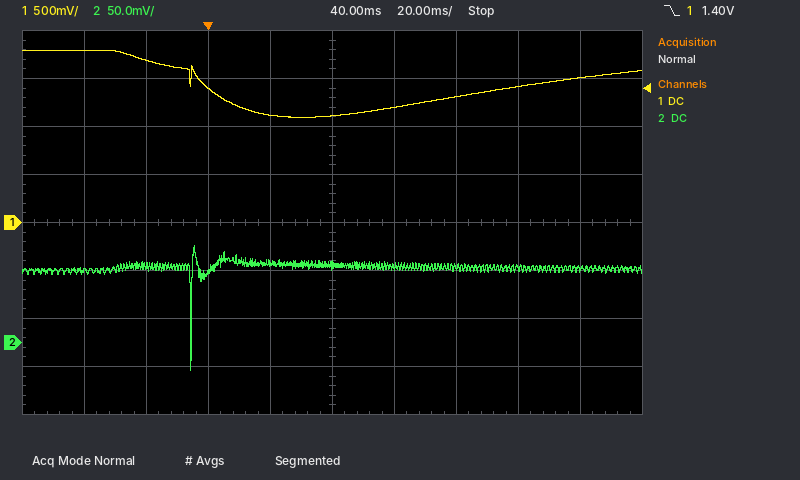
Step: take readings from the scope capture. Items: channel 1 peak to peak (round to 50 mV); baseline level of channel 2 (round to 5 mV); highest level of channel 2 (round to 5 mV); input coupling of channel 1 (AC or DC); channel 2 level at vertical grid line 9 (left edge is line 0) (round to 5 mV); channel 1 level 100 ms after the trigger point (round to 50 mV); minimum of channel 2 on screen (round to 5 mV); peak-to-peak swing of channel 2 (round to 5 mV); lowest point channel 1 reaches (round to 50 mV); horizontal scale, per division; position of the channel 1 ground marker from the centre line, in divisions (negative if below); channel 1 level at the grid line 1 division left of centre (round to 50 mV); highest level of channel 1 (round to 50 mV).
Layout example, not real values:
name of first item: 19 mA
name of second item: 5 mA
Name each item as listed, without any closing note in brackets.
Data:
channel 1 peak to peak: 700 mV
baseline level of channel 2: 80 mV
highest level of channel 2: 100 mV
input coupling of channel 1: DC
channel 2 level at vertical grid line 9 (left edge is line 0): 75 mV
channel 1 level 100 ms after the trigger point: 1.40 V
minimum of channel 2 on screen: -30 mV
peak-to-peak swing of channel 2: 130 mV
lowest point channel 1 reaches: 1.10 V
horizontal scale, per division: 20 ms
position of the channel 1 ground marker from the centre line, in divisions: 0.0 div
channel 1 level at the grid line 1 division left of centre: 1.10 V
highest level of channel 1: 1.80 V
